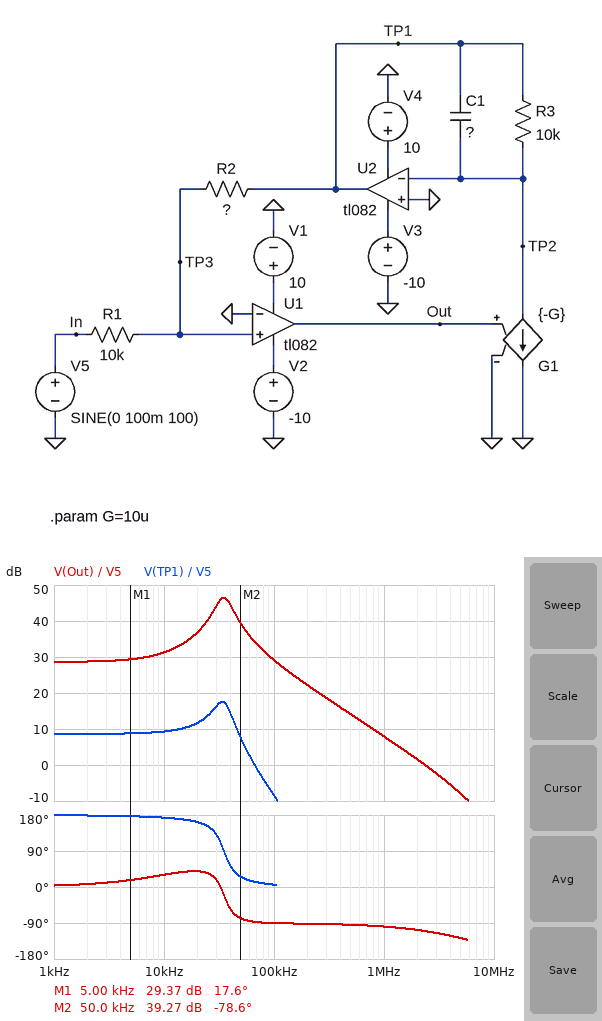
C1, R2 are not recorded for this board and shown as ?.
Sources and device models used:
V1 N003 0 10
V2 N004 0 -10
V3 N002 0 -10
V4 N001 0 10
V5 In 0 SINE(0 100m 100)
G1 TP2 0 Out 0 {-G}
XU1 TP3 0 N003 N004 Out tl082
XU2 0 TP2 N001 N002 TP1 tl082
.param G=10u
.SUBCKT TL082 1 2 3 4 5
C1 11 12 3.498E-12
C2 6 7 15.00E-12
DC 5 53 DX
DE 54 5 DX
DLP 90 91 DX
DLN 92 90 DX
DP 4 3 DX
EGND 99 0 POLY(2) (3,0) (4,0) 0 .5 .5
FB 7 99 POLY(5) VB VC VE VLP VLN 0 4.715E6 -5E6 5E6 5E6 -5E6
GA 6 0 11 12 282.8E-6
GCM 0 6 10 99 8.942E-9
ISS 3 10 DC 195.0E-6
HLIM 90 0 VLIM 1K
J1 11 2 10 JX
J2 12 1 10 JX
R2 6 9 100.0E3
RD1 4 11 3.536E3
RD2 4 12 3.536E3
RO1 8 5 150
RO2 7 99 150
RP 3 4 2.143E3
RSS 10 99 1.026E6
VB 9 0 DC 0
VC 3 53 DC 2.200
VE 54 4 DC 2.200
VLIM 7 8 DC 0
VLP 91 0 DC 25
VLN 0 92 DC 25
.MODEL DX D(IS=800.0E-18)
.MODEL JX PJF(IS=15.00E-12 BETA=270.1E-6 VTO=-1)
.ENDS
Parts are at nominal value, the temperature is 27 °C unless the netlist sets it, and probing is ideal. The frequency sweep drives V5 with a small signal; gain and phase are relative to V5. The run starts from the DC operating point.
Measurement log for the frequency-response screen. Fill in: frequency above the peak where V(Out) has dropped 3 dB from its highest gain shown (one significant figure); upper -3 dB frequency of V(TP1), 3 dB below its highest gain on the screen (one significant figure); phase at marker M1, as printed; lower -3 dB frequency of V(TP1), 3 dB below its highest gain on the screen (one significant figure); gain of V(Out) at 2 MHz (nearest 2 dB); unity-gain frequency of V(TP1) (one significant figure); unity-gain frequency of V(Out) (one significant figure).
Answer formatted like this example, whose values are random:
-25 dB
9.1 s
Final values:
40 kHz
40 kHz
17.6 deg
30 kHz
2 dB
70 kHz
2 MHz
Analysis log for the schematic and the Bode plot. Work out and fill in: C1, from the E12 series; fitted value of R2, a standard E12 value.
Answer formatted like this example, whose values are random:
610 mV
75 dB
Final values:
1.2 nF
27 kΩ
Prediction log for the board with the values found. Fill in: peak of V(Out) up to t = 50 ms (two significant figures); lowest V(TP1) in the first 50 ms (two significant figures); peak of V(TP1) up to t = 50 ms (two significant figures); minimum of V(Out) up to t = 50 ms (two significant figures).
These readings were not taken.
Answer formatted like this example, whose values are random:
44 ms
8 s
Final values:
2.7 V
-270 mV
270 mV
-2.7 V
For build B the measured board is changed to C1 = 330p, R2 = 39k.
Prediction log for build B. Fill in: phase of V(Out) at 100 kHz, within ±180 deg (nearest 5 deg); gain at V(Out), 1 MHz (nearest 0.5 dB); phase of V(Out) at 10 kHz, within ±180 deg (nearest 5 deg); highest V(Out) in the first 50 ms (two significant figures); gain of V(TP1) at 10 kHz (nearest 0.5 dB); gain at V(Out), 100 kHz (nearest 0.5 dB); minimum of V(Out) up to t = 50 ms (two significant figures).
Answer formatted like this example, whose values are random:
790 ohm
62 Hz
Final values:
-80 deg
8.5 dB
5 deg
3.9 V
12.0 dB
31.5 dB
-3.9 V
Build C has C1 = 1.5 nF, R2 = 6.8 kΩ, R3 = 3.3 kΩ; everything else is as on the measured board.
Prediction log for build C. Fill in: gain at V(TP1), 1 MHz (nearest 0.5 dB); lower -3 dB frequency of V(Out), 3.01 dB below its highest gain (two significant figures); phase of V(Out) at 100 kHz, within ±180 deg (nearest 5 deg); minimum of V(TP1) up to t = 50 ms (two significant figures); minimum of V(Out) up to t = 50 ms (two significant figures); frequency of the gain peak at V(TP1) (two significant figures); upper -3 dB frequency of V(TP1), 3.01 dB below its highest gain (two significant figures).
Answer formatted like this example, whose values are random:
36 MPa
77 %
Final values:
-50.5 dB
30 kHz
-85 deg
-68 mV
-2.1 V
41 kHz
55 kHz
